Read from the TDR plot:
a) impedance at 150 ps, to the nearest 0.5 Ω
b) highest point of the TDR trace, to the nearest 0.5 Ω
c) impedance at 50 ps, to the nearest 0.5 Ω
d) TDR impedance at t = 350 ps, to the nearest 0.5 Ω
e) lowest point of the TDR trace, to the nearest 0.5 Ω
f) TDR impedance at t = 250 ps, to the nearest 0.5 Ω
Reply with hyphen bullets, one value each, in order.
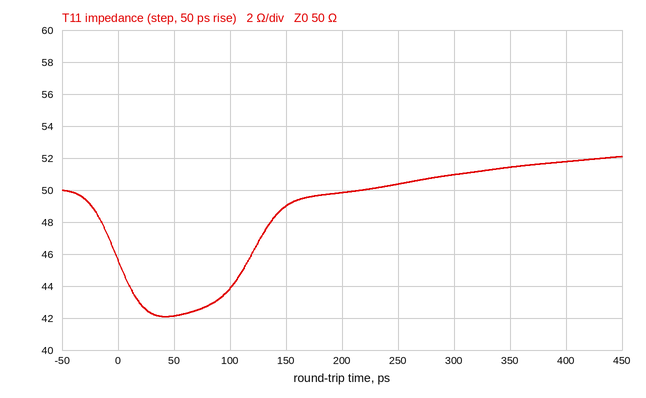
- 49.0 Ω
- 52.0 Ω
- 42.0 Ω
- 51.5 Ω
- 42.0 Ω
- 50.5 Ω
